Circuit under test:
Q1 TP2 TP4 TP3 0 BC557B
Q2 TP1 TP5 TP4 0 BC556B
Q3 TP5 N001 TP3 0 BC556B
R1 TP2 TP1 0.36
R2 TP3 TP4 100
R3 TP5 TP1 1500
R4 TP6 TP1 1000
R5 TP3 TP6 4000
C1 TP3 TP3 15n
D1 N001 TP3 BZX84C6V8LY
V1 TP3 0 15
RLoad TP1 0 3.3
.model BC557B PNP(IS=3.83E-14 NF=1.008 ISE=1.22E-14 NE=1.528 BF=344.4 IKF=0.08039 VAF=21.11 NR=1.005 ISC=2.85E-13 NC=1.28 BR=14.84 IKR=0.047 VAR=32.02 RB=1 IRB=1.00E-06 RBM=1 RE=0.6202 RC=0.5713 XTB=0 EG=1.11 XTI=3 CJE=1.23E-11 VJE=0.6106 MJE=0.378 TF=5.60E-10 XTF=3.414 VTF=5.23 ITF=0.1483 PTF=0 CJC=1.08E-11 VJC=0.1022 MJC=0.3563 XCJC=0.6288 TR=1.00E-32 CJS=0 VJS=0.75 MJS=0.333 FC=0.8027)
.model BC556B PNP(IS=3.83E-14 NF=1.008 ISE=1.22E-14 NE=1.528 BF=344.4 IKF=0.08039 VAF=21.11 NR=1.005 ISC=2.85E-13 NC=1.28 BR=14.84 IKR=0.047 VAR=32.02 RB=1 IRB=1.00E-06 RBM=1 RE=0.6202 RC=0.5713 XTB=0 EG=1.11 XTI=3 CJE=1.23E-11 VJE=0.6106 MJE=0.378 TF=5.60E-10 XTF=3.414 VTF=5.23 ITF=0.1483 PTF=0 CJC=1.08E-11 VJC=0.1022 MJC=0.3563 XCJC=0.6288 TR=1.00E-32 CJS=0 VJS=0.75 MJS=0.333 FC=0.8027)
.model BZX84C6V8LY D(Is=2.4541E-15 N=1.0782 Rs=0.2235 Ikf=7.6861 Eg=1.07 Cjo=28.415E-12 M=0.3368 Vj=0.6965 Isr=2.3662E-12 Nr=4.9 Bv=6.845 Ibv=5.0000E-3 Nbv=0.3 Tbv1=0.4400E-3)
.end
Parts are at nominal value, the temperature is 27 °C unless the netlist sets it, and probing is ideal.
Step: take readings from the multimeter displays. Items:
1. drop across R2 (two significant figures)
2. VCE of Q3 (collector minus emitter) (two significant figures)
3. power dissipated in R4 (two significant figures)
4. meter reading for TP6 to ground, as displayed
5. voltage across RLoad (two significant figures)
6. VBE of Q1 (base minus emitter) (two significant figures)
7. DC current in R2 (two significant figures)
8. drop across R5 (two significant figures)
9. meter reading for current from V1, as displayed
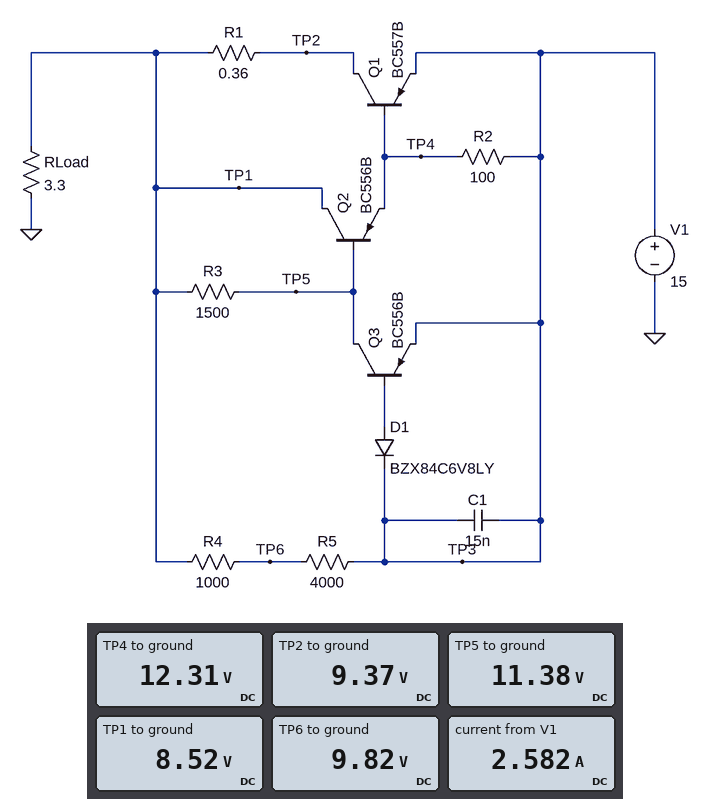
2.7 V
-3.6 V
1.7 mW
9.82 V
8.5 V
-2.7 V
27 mA
5.2 V
2.582 A
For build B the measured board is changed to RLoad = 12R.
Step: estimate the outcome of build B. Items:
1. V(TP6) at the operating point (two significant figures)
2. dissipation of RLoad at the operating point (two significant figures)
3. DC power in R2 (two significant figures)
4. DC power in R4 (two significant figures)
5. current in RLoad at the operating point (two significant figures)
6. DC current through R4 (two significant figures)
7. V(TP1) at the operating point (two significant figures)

13 V
13 W
24 mW
290 µW
1.0 A
540 µA
12 V
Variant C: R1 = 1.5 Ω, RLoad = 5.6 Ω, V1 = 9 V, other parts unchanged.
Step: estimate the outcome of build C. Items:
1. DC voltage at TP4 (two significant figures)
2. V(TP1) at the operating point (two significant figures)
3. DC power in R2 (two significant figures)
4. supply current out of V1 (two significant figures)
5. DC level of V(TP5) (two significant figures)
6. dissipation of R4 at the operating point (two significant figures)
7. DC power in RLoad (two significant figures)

7.4 V
6.1 V
25 mW
1.1 A
6.6 V
340 µW
6.6 W
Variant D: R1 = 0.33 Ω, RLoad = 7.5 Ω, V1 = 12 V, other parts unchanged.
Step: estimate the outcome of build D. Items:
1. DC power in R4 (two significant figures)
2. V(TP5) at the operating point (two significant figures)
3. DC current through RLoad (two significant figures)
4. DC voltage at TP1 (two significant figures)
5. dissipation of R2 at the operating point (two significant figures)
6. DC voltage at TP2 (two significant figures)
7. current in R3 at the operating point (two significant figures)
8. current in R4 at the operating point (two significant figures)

360 µW
9.5 V
1.2 A
9.0 V
28 mW
9.4 V
360 µA
600 µA
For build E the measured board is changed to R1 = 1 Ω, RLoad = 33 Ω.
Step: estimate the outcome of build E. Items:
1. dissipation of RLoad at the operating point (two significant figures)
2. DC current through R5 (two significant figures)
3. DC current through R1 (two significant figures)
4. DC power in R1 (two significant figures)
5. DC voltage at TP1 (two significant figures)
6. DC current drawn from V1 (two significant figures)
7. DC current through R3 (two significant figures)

5.2 W
380 µA
380 mA
140 mW
13 V
400 mA
63 µA
